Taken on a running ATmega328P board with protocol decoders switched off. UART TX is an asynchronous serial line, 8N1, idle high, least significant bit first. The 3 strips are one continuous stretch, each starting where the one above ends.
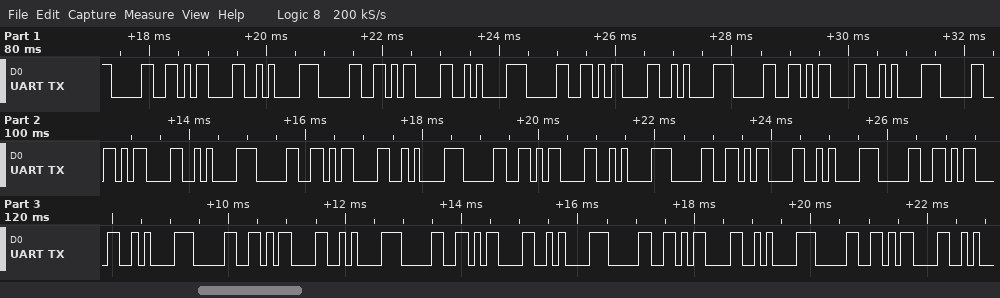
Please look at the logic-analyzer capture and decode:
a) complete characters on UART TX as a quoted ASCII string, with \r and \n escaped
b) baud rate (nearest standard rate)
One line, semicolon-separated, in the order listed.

"0\r\n0\r\n0\r\n0\r\n0\r\n0\r\n0\r\n0\r\n0\r\n0\r\n0\r\n0\r\n0\r"; 9600 baud
